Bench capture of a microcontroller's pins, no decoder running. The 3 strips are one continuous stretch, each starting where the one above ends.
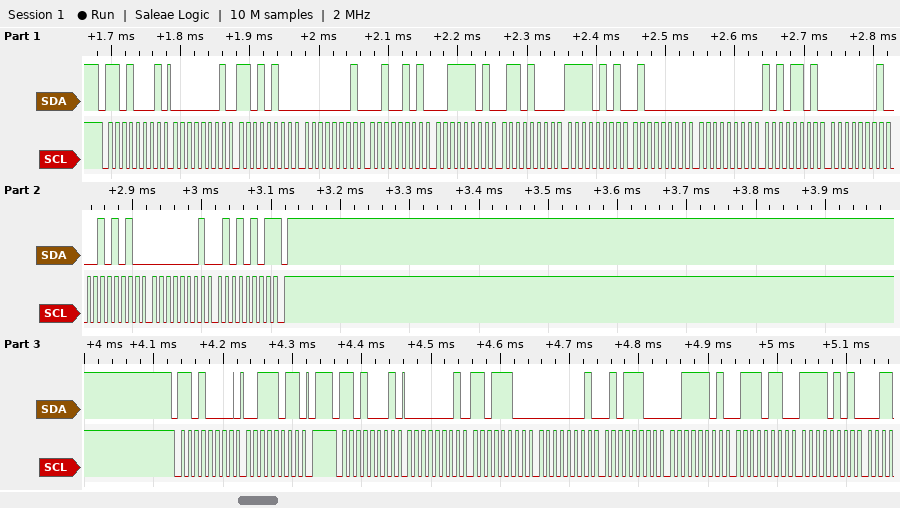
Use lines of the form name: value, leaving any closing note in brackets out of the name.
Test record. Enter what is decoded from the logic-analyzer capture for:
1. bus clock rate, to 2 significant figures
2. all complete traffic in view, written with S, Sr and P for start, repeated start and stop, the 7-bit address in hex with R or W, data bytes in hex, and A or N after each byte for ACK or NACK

bus clock rate, to 2 significant figures: 100 kHz
all complete traffic in view, written with S, Sr and P for start, repeated start and stop, the 7-bit address in hex with R or W, data bytes in hex, and A or N after each byte for ACK or NACK: S 68R A 01 A D4 A 01 A 25 A 3D A 68 A F5 A 40 A 00 A AD A 01 A 2A A 01 A 55 N P S 68W A 3B A P S 68R A 01 A DC A 01 A 5C A 3D A 76 A F5 A
